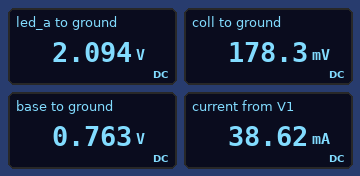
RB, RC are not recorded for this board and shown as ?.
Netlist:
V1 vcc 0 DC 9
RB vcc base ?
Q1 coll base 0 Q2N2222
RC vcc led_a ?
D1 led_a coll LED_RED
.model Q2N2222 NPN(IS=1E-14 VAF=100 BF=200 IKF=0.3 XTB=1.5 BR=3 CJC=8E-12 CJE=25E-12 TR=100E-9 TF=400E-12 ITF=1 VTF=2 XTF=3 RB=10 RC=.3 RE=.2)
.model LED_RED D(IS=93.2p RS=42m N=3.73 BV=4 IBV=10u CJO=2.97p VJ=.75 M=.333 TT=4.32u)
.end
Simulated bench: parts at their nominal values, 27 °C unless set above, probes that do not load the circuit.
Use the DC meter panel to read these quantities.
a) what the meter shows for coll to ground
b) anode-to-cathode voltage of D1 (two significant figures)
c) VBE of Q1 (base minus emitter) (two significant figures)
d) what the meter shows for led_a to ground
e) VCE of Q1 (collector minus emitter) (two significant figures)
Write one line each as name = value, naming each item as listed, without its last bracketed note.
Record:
what the meter shows for coll to ground = 178.3 mV
anode-to-cathode voltage of D1 = 1.9 V
VBE of Q1 (base minus emitter) = 760 mV
what the meter shows for led_a to ground = 2.094 V
VCE of Q1 (collector minus emitter) = 180 mV
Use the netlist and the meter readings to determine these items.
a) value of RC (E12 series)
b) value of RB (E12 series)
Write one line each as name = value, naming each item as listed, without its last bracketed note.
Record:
value of RC = 180 Ω
value of RB = 33 kΩ
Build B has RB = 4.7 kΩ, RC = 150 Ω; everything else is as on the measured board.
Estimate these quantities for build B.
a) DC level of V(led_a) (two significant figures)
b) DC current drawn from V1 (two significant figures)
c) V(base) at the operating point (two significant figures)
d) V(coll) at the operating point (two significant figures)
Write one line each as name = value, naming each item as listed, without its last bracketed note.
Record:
DC level of V(led_a) = 2.0 V
DC current drawn from V1 = 48 mA
V(base) at the operating point = 790 mV
V(coll) at the operating point = 92 mV
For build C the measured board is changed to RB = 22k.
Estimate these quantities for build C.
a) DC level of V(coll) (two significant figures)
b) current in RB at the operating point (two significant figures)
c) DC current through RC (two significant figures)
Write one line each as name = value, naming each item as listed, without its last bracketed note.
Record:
DC level of V(coll) = 140 mV
current in RB at the operating point = 370 µA
DC current through RC = 39 mA
